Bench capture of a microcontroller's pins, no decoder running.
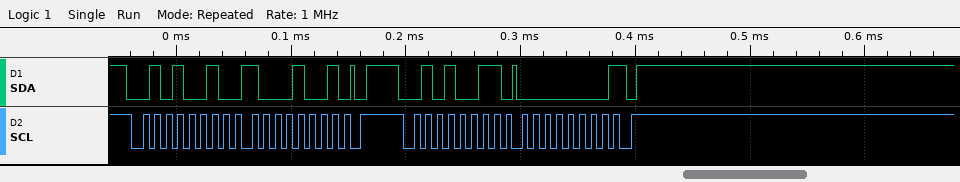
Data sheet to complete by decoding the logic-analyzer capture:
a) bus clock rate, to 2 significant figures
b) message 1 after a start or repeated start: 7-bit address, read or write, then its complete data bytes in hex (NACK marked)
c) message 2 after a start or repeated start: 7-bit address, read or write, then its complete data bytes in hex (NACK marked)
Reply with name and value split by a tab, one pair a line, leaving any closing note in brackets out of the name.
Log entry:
bus clock rate, to 2 significant figures	100 kHz
message 1 after a start or repeated start: 7-bit address, read or write, then its complete data bytes in hex	0x29 write: 89
message 2 after a start or repeated start: 7-bit address, read or write, then its complete data bytes in hex	0x29 read: 00 NACK
